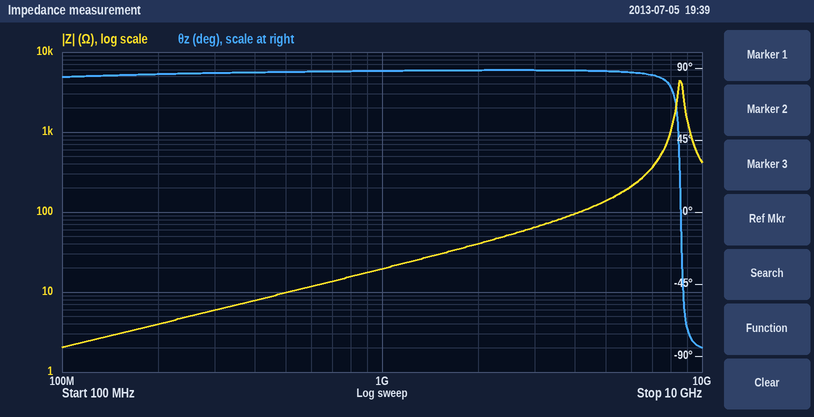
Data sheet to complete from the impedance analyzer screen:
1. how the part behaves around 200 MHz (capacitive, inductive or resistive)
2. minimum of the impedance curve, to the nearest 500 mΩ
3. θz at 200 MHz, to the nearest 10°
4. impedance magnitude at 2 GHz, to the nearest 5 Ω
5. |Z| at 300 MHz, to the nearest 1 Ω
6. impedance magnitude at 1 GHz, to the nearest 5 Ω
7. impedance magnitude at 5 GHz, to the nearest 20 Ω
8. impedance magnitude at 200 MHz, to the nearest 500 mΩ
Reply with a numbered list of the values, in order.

1. inductive
2. 2.0 Ω
3. 90°
4. 40 Ω
5. 6 Ω
6. 20 Ω
7. 140 Ω
8. 4.0 Ω
